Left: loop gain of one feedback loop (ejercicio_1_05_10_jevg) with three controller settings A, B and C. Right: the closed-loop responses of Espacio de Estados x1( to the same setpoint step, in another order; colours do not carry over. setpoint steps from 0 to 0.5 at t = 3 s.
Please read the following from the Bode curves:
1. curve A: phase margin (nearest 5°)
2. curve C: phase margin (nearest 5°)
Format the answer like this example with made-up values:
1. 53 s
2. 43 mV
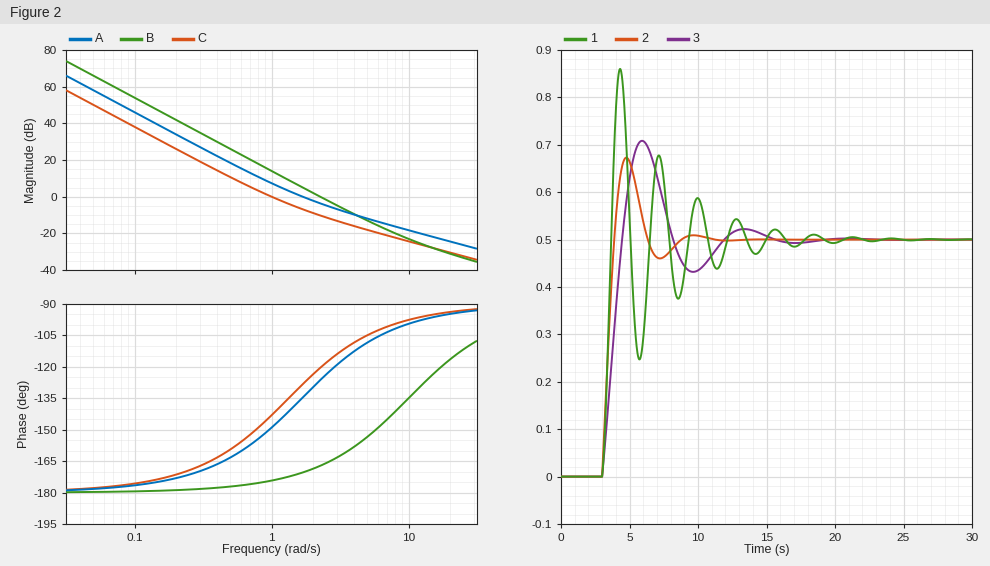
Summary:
1. 45°
2. 35°
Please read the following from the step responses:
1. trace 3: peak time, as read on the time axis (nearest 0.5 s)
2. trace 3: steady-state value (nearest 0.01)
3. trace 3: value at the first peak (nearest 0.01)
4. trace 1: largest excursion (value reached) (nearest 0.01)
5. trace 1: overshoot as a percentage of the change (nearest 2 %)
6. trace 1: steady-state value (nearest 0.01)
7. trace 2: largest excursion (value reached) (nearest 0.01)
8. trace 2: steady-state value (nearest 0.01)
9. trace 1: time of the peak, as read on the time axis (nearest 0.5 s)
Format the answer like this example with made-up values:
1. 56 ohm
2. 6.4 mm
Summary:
1. 6.0 s
2. 0.50
3. 0.71
4. 0.86
5. 72 %
6. 0.50
7. 0.67
8. 0.50
9. 4.5 s
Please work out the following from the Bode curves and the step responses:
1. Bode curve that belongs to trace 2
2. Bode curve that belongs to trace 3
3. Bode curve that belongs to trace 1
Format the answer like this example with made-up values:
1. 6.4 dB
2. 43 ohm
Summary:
1. A
2. C
3. B
